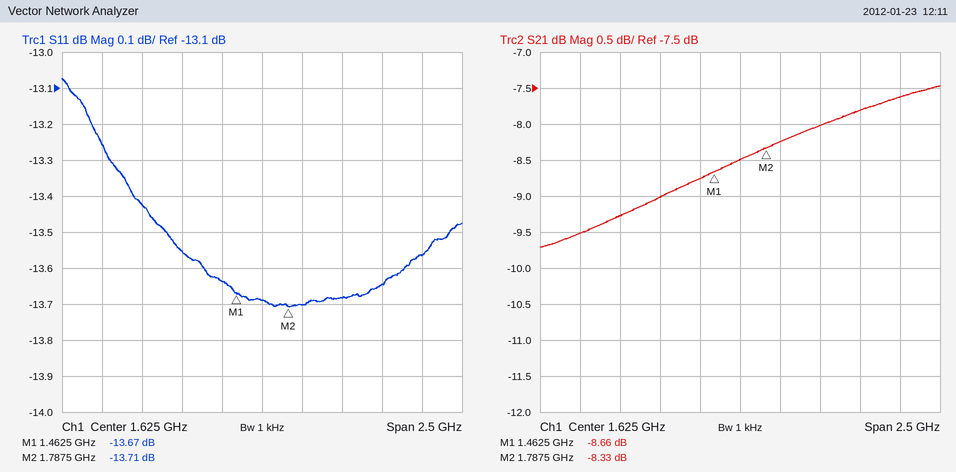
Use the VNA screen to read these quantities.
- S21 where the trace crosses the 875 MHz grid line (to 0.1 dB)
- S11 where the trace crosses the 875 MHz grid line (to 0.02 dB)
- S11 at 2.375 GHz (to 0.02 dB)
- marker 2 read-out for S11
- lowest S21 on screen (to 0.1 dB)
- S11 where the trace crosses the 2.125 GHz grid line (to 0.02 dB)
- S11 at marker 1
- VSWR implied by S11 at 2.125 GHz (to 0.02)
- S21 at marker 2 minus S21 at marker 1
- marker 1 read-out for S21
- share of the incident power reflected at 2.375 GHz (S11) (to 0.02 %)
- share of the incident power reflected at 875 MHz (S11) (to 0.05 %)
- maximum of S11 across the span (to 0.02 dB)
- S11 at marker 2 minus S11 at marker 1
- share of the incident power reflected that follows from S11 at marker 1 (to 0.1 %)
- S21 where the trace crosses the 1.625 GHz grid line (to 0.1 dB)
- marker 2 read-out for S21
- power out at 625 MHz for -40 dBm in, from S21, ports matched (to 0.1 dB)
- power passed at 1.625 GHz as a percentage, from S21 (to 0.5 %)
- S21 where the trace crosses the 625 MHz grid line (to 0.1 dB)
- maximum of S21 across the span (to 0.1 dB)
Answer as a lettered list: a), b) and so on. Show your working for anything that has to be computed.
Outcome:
a) -9.3 dB
b) -13.42 dB
c) -13.64 dB
d) -13.71 dB
e) -9.7 dB
f) -13.68 dB
g) -13.67 dB
h) |Γ| = 10^(-13.68/20) = 0.2070; VSWR = (1 + 0.2070)/(1 − 0.2070) ≈ 1.52
i) -8.33 − (-8.66) = 0.33 dB
j) -8.66 dB
k) 10^(-13.64/10) ≈ 4.33 %, so 4.32 % to the nearest 0.02 %
l) 10^(-13.42/10) ≈ 4.55 %
m) -13.08 dB
n) -13.71 − (-13.67) = -0.04 dB
o) 10^(-13.67/10) ≈ 4.3 %
p) -8.5 dB
q) -8.33 dB
r) -40 dBm + (-9.5 dB) = -49.5 dBm
s) 10^(-8.5/10) ≈ 14.1 %, so 14.0 % to the nearest 0.5 %
t) -9.5 dB
u) -7.5 dB
